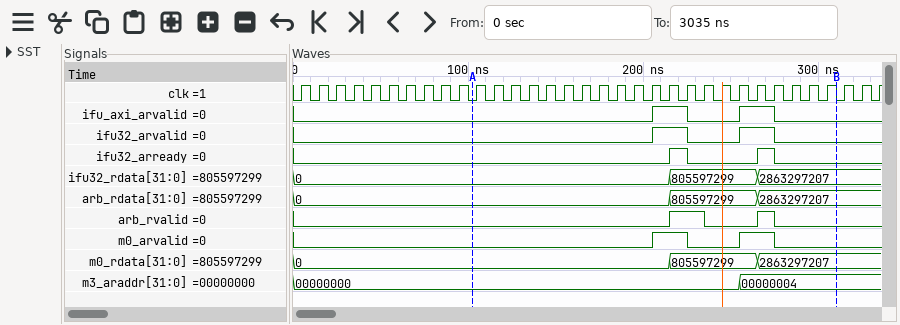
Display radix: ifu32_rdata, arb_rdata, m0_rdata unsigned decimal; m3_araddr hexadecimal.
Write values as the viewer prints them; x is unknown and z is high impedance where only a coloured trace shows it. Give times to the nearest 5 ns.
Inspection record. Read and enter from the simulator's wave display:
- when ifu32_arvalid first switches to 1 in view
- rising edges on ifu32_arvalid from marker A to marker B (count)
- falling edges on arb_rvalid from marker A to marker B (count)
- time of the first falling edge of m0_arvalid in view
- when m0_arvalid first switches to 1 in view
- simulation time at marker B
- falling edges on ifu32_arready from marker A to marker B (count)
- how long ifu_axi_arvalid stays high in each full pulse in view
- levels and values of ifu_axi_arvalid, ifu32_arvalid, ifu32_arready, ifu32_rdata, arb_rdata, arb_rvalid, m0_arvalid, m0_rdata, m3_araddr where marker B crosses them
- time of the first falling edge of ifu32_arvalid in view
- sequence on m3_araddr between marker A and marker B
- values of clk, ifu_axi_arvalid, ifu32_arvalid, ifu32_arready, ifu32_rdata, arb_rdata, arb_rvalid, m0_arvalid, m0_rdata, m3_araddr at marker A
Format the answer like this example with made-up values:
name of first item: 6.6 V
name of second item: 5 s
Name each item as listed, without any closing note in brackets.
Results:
when ifu32_arvalid first switches to 1 in view: 205 ns
rising edges on ifu32_arvalid from marker A to marker B: 2
falling edges on arb_rvalid from marker A to marker B: 2
time of the first falling edge of m0_arvalid in view: 225 ns
when m0_arvalid first switches to 1 in view: 205 ns
simulation time at marker B: 310 ns
falling edges on ifu32_arready from marker A to marker B: 2
how long ifu_axi_arvalid stays high in each full pulse in view: 20 ns, 20 ns
levels and values of ifu_axi_arvalid, ifu32_arvalid, ifu32_arready, ifu32_rdata, arb_rdata, arb_rvalid, m0_arvalid, m0_rdata, m3_araddr where marker B crosses them: ifu_axi_arvalid=0, ifu32_arvalid=0, ifu32_arready=0, ifu32_rdata=2863297207, arb_rdata=2863297207, arb_rvalid=0, m0_arvalid=0, m0_rdata=2863297207, m3_araddr=00000004
time of the first falling edge of ifu32_arvalid in view: 225 ns
sequence on m3_araddr between marker A and marker B: 00000000, 00000004
values of clk, ifu_axi_arvalid, ifu32_arvalid, ifu32_arready, ifu32_rdata, arb_rdata, arb_rvalid, m0_arvalid, m0_rdata, m3_araddr at marker A: clk=0, ifu_axi_arvalid=0, ifu32_arvalid=0, ifu32_arready=0, ifu32_rdata=0, arb_rdata=0, arb_rvalid=0, m0_arvalid=0, m0_rdata=0, m3_araddr=00000000
